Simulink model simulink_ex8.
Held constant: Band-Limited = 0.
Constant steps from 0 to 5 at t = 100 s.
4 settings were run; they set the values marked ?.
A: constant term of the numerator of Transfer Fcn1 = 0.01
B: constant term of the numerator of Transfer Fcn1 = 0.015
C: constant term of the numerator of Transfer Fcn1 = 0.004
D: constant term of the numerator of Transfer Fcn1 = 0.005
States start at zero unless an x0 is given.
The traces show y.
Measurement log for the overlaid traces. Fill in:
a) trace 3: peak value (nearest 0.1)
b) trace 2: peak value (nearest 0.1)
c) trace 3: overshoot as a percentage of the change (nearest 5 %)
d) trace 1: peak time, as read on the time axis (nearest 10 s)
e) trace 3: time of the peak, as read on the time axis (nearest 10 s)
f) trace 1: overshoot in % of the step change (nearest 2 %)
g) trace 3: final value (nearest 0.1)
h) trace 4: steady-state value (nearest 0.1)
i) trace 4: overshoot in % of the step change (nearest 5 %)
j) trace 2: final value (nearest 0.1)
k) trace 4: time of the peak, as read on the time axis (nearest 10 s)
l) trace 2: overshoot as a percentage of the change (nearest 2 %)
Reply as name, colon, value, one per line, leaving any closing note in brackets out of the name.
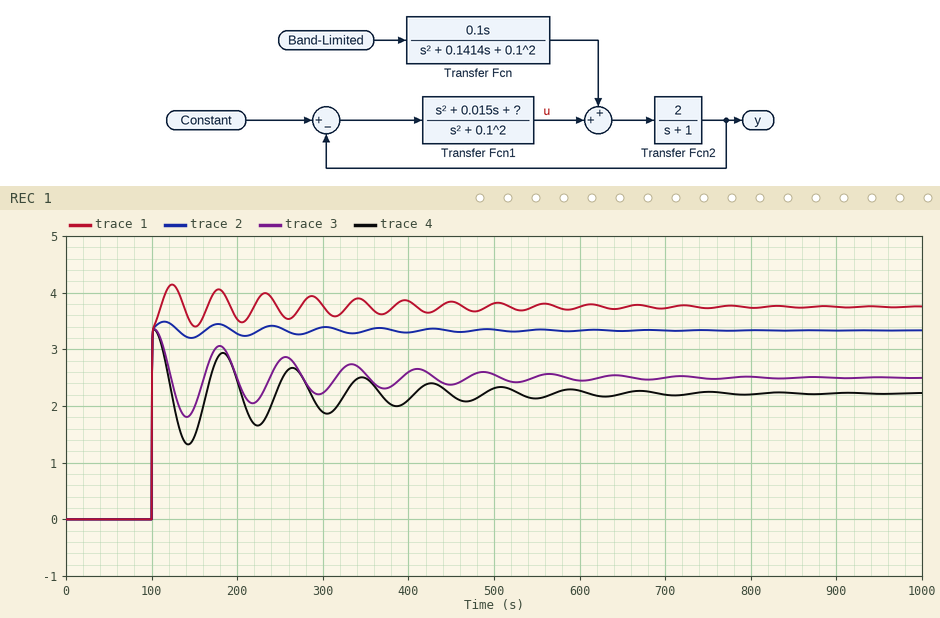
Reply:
trace 3: peak value: 3.4
trace 2: peak value: 3.5
trace 3: overshoot as a percentage of the change: 35 %
trace 1: peak time, as read on the time axis: 120 s
trace 3: time of the peak, as read on the time axis: 100 s
trace 1: overshoot in % of the step change: 10 %
trace 3: final value: 2.5
trace 4: steady-state value: 2.2
trace 4: overshoot in % of the step change: 50 %
trace 2: final value: 3.3
trace 4: time of the peak, as read on the time axis: 100 s
trace 2: overshoot as a percentage of the change: 4 %
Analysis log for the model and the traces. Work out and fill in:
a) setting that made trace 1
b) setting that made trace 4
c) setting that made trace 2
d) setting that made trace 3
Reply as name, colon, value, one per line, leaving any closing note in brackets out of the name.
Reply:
setting that made trace 1: B
setting that made trace 4: C
setting that made trace 2: A
setting that made trace 3: D
